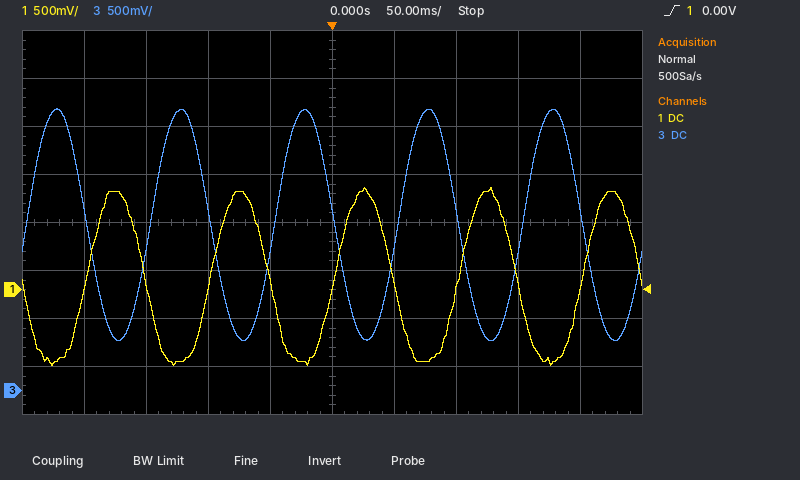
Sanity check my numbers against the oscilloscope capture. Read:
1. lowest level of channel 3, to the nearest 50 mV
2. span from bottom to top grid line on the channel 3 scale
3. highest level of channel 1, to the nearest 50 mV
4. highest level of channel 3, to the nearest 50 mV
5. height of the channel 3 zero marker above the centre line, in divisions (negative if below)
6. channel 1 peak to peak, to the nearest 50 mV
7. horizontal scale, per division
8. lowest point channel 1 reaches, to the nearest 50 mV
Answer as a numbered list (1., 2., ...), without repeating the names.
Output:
1. 500 mV
2. 4 V
3. 1.05 V
4. 2.95 V
5. -3.5 div
6. 1.85 V
7. 50 ms
8. -800 mV
